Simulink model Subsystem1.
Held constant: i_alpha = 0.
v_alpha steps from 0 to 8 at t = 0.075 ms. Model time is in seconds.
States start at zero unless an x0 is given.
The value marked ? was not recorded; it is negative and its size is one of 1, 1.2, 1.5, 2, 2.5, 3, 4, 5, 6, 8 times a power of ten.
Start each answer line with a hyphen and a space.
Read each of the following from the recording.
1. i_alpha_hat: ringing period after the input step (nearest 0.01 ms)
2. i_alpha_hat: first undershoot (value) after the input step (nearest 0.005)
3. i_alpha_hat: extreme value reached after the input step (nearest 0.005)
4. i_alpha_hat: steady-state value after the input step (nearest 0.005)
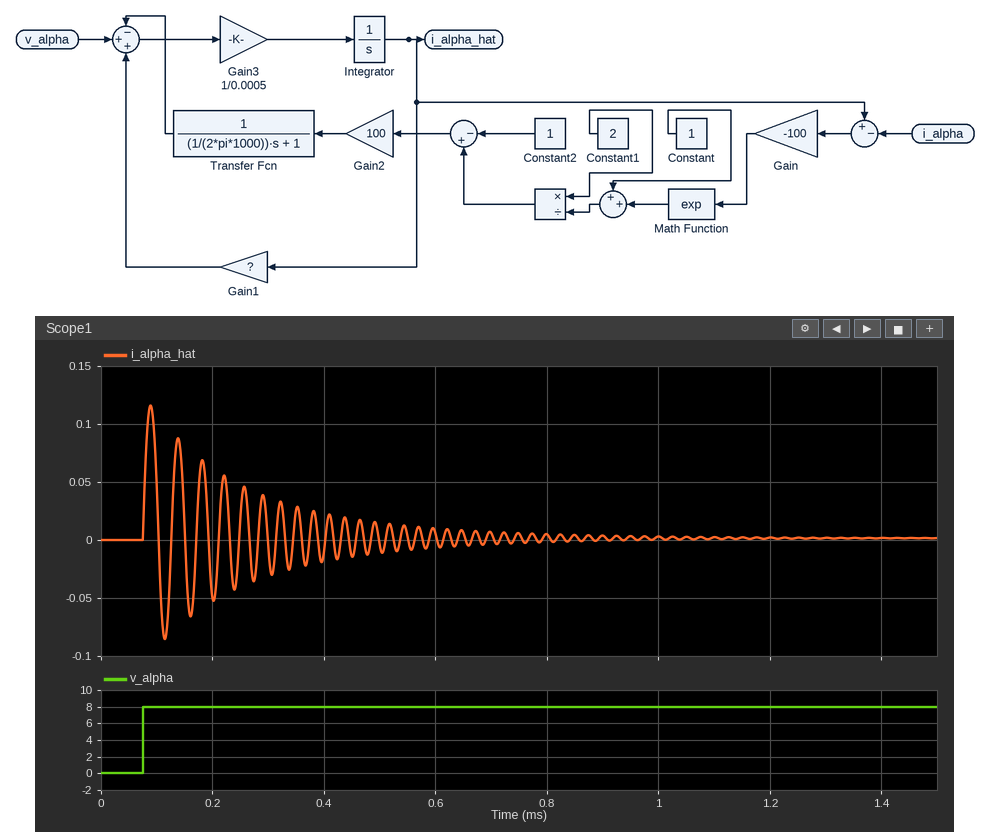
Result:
- 0.05 ms
- -0.085
- 0.115
- 0.000
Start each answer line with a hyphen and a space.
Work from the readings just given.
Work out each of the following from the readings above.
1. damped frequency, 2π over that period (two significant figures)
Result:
- 130 rad/ms
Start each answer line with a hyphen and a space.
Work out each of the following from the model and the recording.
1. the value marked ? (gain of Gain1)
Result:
- -1.2
